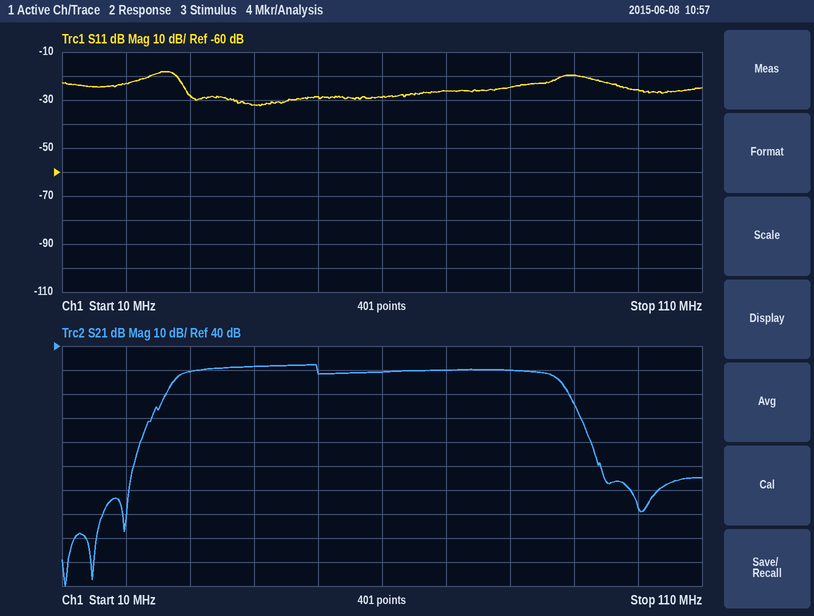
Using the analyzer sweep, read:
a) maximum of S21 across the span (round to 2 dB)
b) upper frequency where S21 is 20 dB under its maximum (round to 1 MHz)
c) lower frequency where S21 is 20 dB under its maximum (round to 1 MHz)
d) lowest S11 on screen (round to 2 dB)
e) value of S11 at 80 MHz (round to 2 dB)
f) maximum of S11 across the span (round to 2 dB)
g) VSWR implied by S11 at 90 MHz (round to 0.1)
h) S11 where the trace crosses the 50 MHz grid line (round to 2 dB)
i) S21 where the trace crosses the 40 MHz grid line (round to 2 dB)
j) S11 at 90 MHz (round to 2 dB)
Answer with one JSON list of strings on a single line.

["32 dB", "91 MHz", "24 MHz", "-32 dB", "-24 dB", "-18 dB", "1.2", "-28 dB", "32 dB", "-20 dB"]
